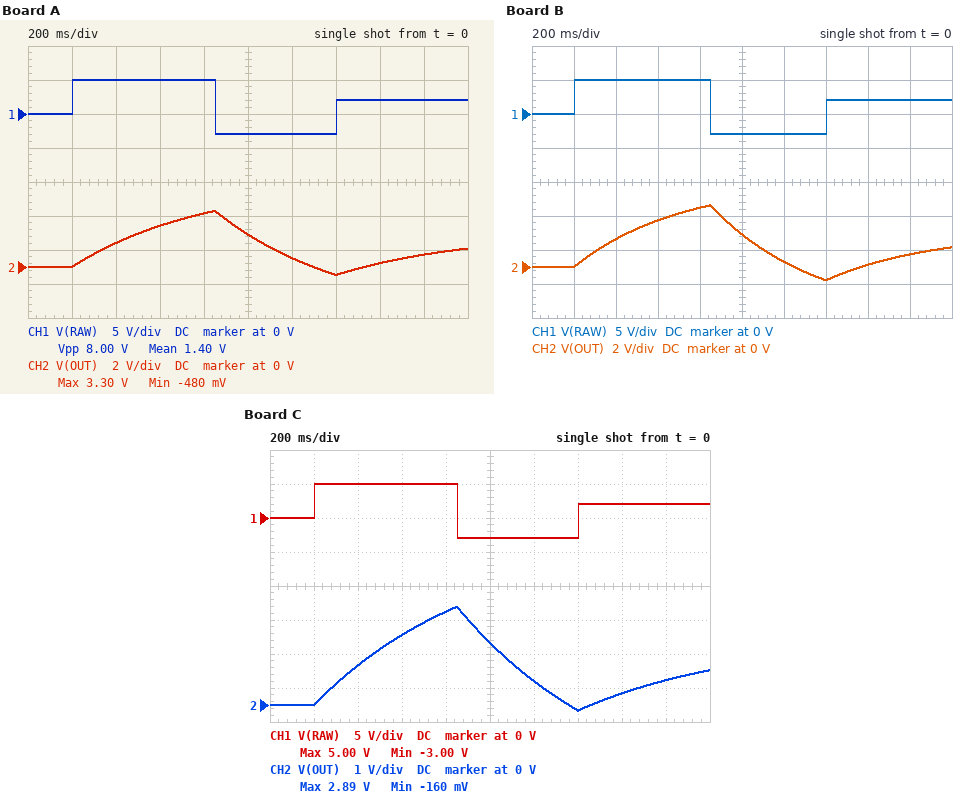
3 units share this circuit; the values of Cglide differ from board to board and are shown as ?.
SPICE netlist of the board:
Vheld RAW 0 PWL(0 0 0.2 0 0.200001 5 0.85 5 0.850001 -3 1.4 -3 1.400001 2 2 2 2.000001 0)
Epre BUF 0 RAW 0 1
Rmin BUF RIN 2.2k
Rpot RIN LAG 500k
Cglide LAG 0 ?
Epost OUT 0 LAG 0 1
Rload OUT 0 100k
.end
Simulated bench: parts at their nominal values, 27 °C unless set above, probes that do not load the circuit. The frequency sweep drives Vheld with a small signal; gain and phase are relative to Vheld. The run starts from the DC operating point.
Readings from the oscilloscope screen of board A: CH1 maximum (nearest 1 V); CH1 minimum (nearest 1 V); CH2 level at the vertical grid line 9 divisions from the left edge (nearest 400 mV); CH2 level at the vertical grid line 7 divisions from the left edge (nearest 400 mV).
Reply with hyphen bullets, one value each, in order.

- 5 V
- -3 V
- 800 mV
- -400 mV
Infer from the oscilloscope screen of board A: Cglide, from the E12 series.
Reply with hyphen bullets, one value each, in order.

- 1.2 µF
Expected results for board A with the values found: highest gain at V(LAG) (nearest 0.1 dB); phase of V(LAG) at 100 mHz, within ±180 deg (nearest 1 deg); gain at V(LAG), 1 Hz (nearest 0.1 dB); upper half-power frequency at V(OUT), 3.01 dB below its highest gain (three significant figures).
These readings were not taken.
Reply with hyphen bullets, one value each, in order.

- 0 dB
- -21 deg
- -11.9 dB
- 264 mHz
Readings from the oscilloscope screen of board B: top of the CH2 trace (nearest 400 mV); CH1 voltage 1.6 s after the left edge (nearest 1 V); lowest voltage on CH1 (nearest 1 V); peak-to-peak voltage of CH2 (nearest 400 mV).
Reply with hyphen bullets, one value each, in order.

- 3.6 V
- 2 V
- -3 V
- 4.4 V
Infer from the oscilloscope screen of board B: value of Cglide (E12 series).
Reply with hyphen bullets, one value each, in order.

- 1 µF
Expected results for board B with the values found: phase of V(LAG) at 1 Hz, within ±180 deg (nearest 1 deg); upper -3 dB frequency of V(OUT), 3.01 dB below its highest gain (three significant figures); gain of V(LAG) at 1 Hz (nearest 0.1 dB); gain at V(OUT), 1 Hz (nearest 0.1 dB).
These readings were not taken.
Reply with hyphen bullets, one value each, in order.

- -72 deg
- 317 mHz
- -10.4 dB
- -10.4 dB
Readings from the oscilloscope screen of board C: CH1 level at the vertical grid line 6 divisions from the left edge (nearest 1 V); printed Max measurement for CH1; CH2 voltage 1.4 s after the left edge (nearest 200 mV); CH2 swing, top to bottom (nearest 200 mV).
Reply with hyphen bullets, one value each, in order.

- -3 V
- 5.00 V
- -200 mV
- 3.0 V
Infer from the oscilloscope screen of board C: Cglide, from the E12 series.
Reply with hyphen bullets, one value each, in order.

- 1.5 µF
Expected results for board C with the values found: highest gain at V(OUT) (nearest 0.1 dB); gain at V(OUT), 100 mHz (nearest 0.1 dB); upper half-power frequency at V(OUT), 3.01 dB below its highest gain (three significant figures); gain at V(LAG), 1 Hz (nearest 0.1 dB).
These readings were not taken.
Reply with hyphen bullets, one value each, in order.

- 0 dB
- -0.9 dB
- 211 mHz
- -13.7 dB
